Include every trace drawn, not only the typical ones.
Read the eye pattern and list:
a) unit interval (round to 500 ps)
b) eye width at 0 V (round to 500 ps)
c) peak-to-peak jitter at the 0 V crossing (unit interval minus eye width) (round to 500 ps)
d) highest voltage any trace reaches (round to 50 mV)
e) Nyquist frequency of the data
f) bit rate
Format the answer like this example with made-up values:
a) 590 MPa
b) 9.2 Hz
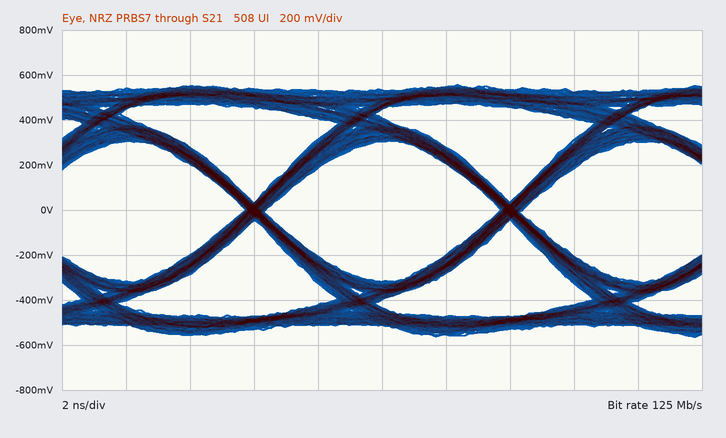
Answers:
a) 8.0 ns
b) 7.5 ns
c) 500 ps
d) 550 mV
e) 62.5 MHz
f) 125 Mb/s
